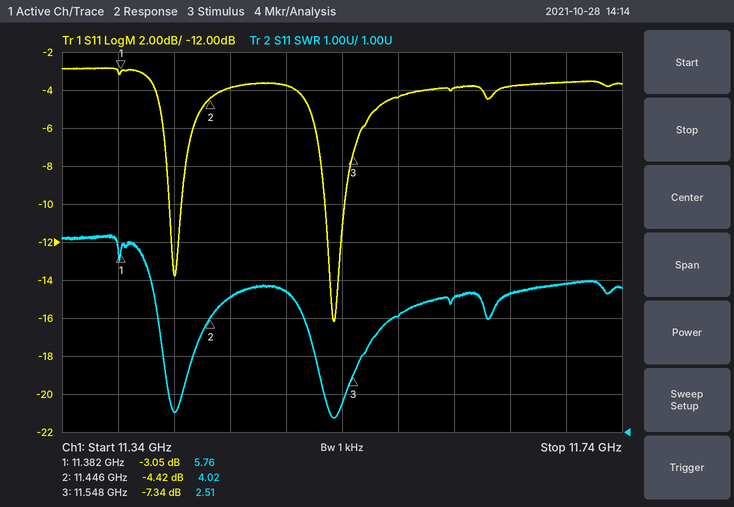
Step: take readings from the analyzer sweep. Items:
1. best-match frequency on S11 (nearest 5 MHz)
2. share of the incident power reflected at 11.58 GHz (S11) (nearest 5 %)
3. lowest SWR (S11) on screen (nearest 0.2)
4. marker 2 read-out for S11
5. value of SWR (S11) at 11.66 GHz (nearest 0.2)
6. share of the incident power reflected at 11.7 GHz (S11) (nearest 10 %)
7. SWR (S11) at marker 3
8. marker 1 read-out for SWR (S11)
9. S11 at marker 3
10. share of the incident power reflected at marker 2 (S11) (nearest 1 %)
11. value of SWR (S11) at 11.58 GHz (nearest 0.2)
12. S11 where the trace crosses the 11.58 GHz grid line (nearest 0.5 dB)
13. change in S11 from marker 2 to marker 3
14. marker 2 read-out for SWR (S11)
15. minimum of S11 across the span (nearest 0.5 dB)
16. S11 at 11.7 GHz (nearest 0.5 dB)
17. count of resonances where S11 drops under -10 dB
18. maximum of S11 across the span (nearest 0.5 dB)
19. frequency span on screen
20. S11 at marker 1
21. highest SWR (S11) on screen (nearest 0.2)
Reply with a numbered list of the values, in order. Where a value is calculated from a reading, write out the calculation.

1. 11.535 GHz
2. 10^(-4.5/10) ≈ 35 %
3. 1.4
4. -4.42 dB
5. 4.6
6. 10^(-3.5/10) ≈ 44.7 %, so 40 % to the nearest 10 %
7. 2.51
8. 5.76
9. -7.34 dB
10. 10^(-4.42/10) ≈ 36 %
11. 4.0
12. -4.5 dB
13. -7.34 − (-4.42) = -2.92 dB
14. 4.02
15. -16.0 dB
16. -3.5 dB
17. 2
18. -3.0 dB
19. 400 MHz
20. -3.05 dB
21. 6.2
